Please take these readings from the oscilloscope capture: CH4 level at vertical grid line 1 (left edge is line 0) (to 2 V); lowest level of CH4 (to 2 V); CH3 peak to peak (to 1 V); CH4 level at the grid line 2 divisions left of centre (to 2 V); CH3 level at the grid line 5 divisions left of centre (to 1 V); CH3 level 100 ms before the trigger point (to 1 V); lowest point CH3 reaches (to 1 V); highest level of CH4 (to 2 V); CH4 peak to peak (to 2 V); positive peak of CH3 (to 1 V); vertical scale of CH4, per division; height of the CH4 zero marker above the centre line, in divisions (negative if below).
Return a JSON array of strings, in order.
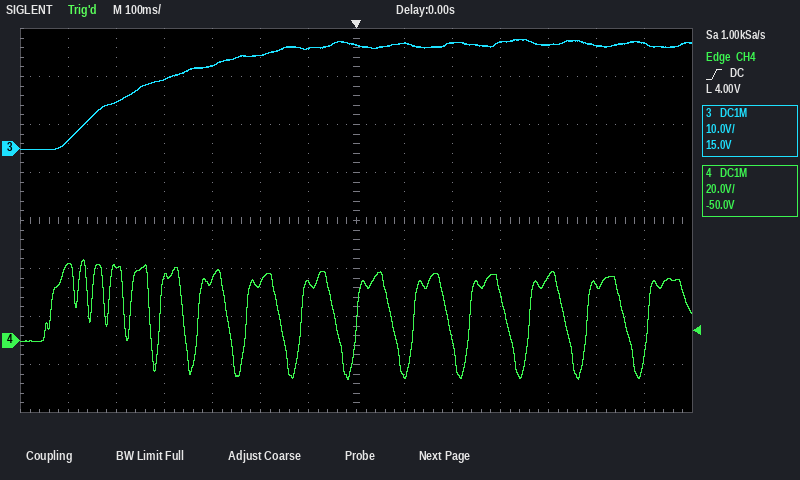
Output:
["32 V", "-16 V", "23 V", "24 V", "10 V", "21 V", "0 V", "34 V", "50 V", "23 V", "20 V", "-2.5 div"]
